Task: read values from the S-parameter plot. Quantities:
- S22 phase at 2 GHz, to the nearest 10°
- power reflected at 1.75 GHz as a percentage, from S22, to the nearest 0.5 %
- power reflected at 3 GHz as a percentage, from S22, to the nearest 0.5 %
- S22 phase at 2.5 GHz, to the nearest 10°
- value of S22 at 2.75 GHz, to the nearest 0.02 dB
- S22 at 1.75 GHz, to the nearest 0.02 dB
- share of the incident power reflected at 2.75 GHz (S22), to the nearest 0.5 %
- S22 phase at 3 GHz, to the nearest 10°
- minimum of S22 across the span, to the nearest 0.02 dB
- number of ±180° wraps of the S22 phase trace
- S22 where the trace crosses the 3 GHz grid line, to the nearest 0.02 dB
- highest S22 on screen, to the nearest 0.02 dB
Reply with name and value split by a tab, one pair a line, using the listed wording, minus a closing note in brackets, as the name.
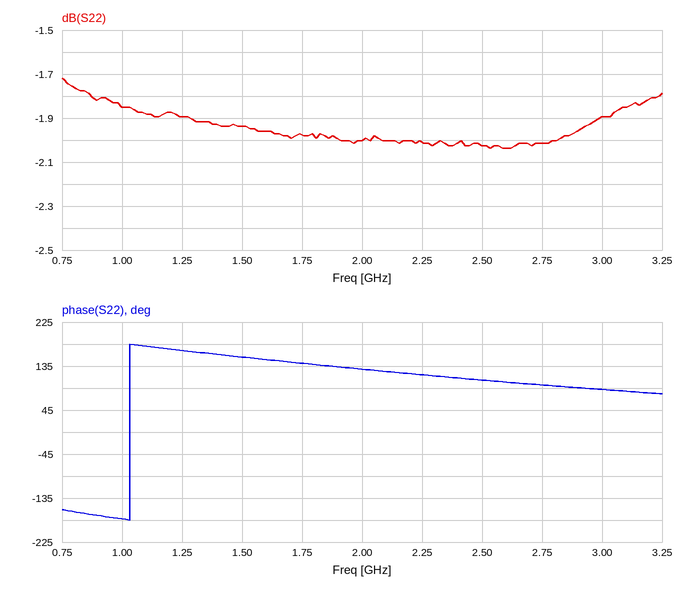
S22 phase at 2 GHz, to the nearest 10°	130°
power reflected at 1.75 GHz as a percentage, from S22, to the nearest 0.5 %	63.5 %
power reflected at 3 GHz as a percentage, from S22, to the nearest 0.5 %	64.5 %
S22 phase at 2.5 GHz, to the nearest 10°	110°
value of S22 at 2.75 GHz, to the nearest 0.02 dB	-2.02 dB
S22 at 1.75 GHz, to the nearest 0.02 dB	-1.98 dB
share of the incident power reflected at 2.75 GHz (S22), to the nearest 0.5 %	63.0 %
S22 phase at 3 GHz, to the nearest 10°	90°
minimum of S22 across the span, to the nearest 0.02 dB	-2.04 dB
number of ±180° wraps of the S22 phase trace	1
S22 where the trace crosses the 3 GHz grid line, to the nearest 0.02 dB	-1.90 dB
highest S22 on screen, to the nearest 0.02 dB	-1.72 dB
